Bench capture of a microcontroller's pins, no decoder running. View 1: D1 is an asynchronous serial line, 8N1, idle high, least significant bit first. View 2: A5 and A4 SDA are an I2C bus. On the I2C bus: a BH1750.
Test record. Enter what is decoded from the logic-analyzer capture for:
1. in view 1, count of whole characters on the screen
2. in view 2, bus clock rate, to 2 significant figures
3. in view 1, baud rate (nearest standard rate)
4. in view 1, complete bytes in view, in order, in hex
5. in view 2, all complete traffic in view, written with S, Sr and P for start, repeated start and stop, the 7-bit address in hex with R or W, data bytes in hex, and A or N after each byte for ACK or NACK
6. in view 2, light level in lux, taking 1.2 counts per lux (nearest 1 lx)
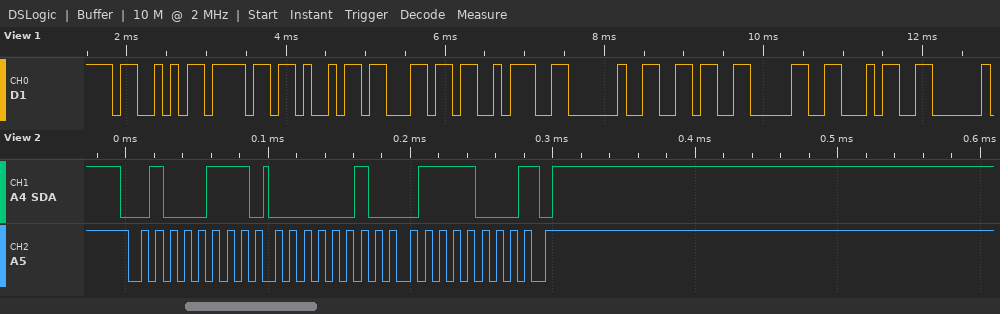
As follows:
9
100 kHz
9600 baud
0x53 0x6F 0x69 0x6C 0x3A 0x20 0x36 0x30 0x34
S 23R A 02 A 78 N P
527 lx
